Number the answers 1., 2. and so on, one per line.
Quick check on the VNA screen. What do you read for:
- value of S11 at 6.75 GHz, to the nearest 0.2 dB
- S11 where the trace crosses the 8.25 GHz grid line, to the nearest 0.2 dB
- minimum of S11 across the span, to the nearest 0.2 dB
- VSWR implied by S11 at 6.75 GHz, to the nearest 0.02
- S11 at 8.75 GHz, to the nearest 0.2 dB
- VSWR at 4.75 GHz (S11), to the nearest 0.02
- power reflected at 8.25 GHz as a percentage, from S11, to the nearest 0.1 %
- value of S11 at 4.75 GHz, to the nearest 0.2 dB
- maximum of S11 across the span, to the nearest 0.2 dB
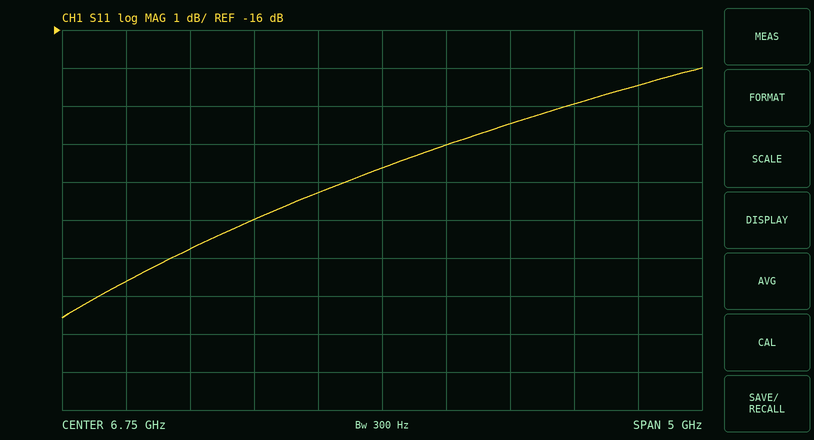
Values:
1. -19.6 dB
2. -18.0 dB
3. -23.6 dB
4. 1.24
5. -17.4 dB
6. 1.16
7. 1.6 %
8. -22.6 dB
9. -17.0 dB
